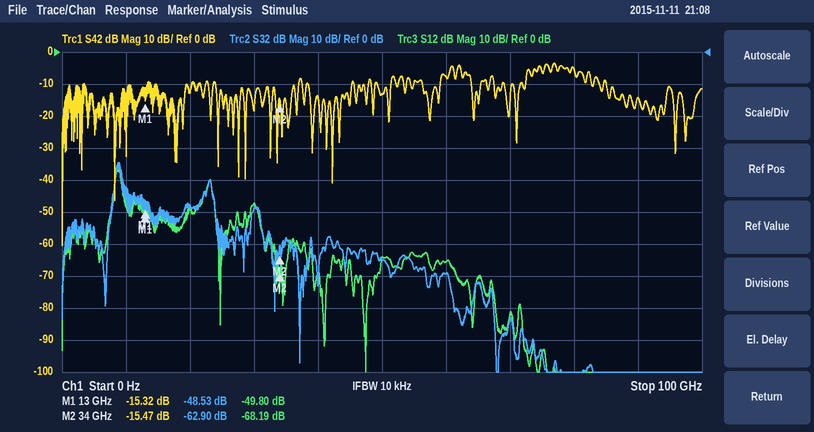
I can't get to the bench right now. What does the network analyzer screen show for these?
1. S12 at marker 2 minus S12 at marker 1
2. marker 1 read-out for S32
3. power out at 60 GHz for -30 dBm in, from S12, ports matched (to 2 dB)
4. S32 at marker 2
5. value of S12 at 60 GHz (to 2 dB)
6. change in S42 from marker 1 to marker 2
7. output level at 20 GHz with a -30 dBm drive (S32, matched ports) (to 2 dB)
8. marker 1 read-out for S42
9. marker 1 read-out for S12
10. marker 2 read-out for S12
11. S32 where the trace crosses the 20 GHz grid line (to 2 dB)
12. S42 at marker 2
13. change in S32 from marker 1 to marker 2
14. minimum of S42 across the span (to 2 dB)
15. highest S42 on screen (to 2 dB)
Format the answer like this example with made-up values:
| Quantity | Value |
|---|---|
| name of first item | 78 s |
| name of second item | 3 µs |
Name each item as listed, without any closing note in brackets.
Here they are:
| Quantity | Value |
|---|---|
| S12 at marker 2 minus S12 at marker 1 | -18.39 dB |
| marker 1 read-out for S32 | -48.53 dB |
| power out at 60 GHz for -30 dBm in, from S12, ports matched | -96 dBm |
| S32 at marker 2 | -62.90 dB |
| value of S12 at 60 GHz | -66 dB |
| change in S42 from marker 1 to marker 2 | -0.15 dB |
| output level at 20 GHz with a -30 dBm drive (S32, matched ports) | -78 dBm |
| marker 1 read-out for S42 | -15.32 dB |
| marker 1 read-out for S12 | -49.80 dB |
| marker 2 read-out for S12 | -68.19 dB |
| S32 where the trace crosses the 20 GHz grid line | -48 dB |
| S42 at marker 2 | -15.47 dB |
| change in S32 from marker 1 to marker 2 | -14.37 dB |
| minimum of S42 across the span | -60 dB |
| highest S42 on screen | -4 dB |
